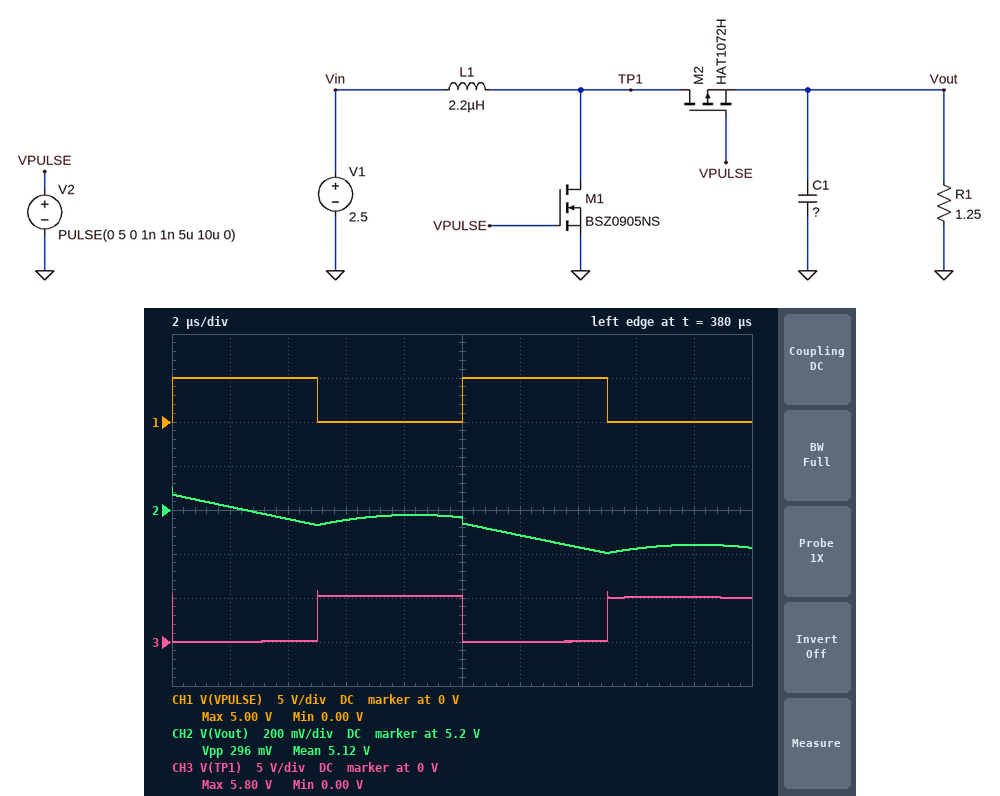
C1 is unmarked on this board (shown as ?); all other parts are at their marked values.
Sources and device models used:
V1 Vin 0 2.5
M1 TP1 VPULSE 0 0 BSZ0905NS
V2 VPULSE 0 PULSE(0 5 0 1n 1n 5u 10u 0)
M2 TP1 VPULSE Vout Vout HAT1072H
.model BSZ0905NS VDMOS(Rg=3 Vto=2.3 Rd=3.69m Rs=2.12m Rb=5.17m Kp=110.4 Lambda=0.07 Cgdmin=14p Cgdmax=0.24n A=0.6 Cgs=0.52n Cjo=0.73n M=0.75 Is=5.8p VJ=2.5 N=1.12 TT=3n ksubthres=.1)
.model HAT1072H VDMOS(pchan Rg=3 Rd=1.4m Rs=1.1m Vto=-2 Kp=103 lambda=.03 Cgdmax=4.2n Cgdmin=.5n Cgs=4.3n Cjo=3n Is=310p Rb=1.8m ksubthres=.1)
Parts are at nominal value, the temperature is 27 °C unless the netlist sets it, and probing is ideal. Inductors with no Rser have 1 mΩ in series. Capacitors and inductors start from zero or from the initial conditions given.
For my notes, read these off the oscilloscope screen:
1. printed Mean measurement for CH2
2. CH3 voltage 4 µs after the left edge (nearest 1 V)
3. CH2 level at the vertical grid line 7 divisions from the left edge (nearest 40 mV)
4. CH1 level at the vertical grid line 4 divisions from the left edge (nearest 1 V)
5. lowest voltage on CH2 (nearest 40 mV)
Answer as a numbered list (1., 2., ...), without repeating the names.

1. 5.12 V
2. 0 V
3. 5.04 V
4. 0 V
5. 5.00 V
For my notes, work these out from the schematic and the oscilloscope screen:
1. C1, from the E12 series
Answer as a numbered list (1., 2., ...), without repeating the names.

1. 150 µF
